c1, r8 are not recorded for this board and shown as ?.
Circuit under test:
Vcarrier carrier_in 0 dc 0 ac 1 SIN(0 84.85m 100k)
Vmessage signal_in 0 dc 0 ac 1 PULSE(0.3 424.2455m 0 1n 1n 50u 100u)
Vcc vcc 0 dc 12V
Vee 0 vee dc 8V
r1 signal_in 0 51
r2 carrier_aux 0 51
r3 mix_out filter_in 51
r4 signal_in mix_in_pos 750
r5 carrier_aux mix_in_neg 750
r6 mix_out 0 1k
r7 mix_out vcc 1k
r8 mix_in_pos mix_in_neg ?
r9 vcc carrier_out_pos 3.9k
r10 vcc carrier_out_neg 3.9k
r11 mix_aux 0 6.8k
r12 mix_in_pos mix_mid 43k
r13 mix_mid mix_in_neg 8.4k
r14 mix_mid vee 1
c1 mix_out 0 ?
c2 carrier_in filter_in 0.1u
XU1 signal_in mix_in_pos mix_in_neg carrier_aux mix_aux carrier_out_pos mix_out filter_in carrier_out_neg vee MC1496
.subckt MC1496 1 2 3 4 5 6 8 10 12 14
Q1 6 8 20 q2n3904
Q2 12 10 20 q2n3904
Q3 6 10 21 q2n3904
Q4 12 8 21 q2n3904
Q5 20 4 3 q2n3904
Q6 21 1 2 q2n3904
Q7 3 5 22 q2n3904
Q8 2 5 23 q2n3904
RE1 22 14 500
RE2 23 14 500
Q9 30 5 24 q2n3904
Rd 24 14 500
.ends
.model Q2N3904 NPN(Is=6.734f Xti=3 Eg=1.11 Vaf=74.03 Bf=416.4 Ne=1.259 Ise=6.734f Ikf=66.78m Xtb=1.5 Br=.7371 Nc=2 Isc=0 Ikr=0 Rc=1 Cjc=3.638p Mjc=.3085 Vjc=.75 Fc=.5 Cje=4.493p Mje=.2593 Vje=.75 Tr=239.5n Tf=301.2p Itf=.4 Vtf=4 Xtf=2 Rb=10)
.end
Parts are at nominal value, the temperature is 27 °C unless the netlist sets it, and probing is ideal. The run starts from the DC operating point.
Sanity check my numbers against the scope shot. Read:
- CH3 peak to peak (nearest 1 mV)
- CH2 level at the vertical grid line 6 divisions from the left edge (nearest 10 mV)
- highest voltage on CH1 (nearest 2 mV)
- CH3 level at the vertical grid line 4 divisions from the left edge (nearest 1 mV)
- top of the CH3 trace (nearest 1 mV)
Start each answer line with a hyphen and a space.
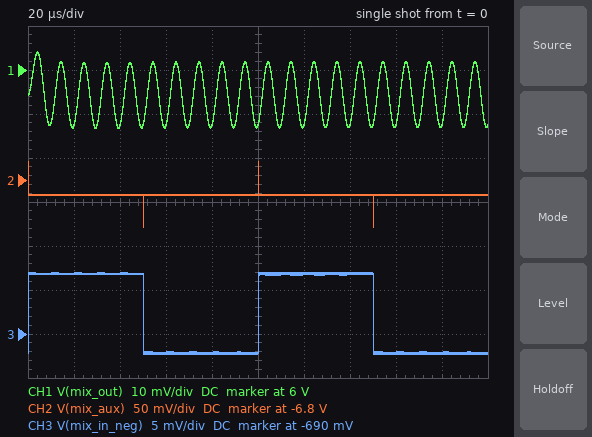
- 9 mV
- -6.82 V
- 6.004 V
- -692 mV
- -683 mV
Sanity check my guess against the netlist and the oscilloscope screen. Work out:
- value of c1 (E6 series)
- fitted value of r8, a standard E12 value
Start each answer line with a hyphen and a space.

- 330 nF
- 680 Ω
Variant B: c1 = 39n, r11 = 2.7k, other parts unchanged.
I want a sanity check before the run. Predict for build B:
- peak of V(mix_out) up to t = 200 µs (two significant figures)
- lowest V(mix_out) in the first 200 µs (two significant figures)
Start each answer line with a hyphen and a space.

- 5.9 V
- 5.8 V
